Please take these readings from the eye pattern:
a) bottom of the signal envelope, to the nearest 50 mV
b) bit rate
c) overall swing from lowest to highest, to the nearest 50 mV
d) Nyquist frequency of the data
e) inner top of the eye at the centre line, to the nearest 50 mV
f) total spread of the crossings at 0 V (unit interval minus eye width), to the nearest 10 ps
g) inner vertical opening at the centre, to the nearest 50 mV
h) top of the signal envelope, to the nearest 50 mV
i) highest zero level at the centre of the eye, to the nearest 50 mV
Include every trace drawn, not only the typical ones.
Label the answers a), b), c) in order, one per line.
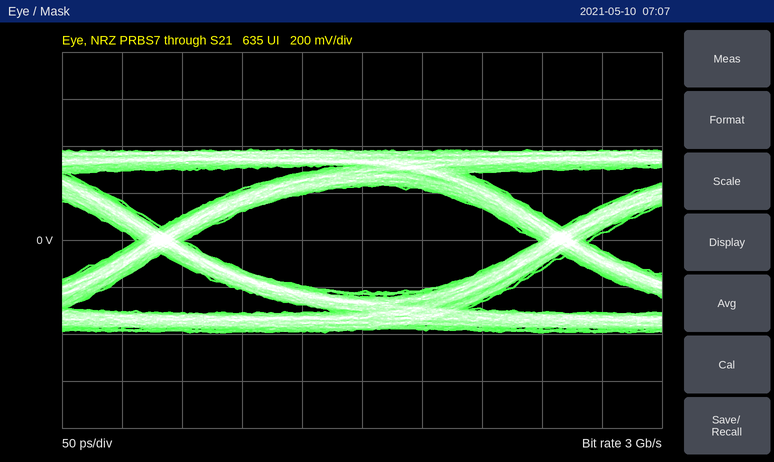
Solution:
a) -400 mV
b) 3 Gb/s
c) 800 mV
d) 1.5 GHz
e) 250 mV
f) 40 ps
g) 450 mV
h) 400 mV
i) -200 mV
